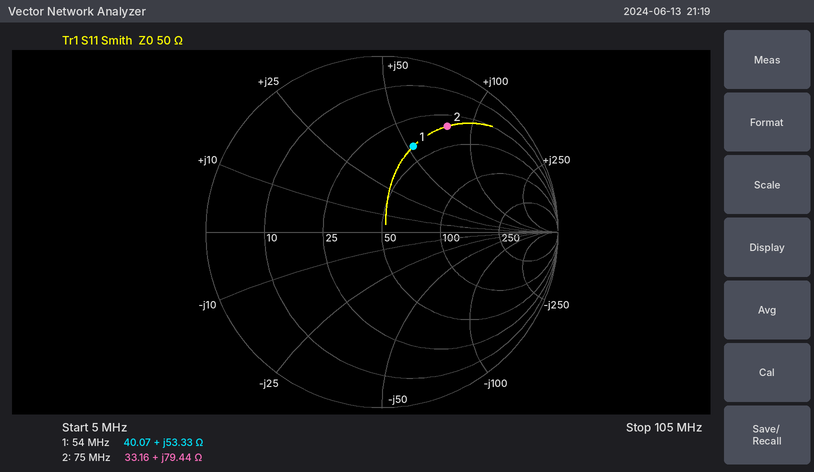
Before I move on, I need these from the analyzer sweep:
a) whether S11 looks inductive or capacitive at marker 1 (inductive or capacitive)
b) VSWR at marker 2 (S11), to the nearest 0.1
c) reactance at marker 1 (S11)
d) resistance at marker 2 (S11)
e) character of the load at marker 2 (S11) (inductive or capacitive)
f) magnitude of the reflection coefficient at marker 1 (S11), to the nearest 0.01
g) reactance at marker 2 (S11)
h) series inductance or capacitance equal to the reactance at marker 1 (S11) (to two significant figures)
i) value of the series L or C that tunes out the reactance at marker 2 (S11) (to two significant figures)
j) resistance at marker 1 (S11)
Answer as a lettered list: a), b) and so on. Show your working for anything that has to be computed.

a) inductive
b) 5.8
c) +53.33 Ω
d) 33.16 Ω
e) inductive
f) 0.52
g) +79.44 Ω
h) L = 53.33 Ω/(2π × 54 MHz) ≈ 157 nH, so 160 nH to two significant figures
i) C = 1/(2π × 75 MHz × 79.44 Ω) ≈ 27 pF
j) 40.07 Ω
